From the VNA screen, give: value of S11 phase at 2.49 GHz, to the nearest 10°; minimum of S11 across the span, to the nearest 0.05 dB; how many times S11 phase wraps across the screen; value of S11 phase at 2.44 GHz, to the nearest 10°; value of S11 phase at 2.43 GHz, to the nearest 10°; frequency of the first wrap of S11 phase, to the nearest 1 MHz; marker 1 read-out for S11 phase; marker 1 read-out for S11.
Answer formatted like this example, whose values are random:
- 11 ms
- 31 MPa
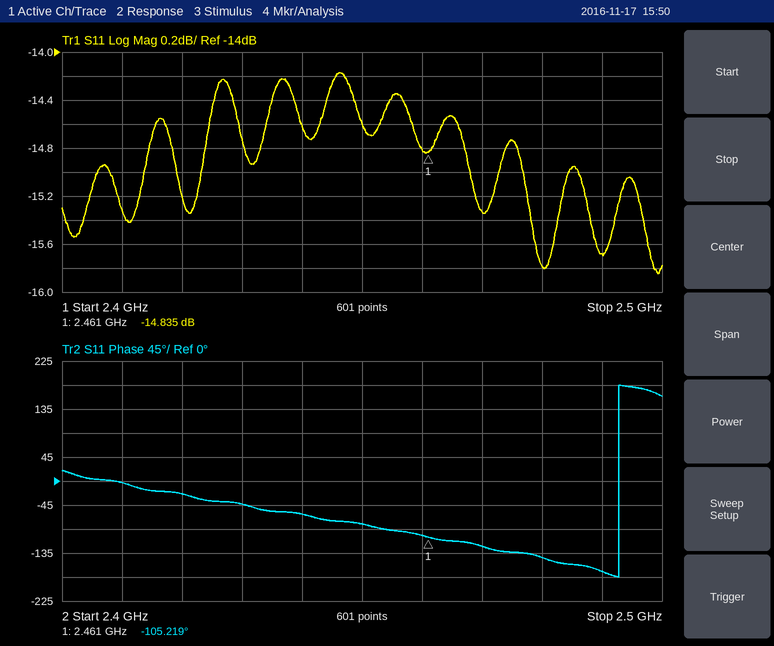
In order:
- -170°
- -15.85 dB
- 1
- -60°
- -40°
- 2.493 GHz
- -105.219°
- -14.835 dB
